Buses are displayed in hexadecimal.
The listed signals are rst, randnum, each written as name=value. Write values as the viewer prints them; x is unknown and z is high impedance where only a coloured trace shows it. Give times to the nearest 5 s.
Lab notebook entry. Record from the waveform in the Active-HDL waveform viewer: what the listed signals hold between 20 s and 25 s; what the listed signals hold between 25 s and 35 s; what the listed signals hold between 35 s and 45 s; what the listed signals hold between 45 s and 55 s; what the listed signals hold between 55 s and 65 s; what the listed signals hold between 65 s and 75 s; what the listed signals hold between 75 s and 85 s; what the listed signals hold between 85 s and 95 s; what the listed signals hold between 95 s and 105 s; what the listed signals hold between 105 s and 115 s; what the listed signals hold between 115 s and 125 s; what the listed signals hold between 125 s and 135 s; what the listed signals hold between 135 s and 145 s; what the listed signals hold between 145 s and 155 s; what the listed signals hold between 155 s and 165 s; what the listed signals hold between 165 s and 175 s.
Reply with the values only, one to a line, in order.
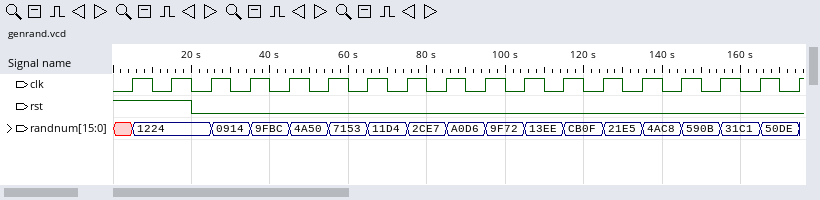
rst=0, randnum=1224
rst=0, randnum=0914
rst=0, randnum=9FBC
rst=0, randnum=4A50
rst=0, randnum=7153
rst=0, randnum=11D4
rst=0, randnum=2CE7
rst=0, randnum=A0D6
rst=0, randnum=9F72
rst=0, randnum=13EE
rst=0, randnum=CB0F
rst=0, randnum=21E5
rst=0, randnum=4AC8
rst=0, randnum=590B
rst=0, randnum=31C1
rst=0, randnum=50DE
